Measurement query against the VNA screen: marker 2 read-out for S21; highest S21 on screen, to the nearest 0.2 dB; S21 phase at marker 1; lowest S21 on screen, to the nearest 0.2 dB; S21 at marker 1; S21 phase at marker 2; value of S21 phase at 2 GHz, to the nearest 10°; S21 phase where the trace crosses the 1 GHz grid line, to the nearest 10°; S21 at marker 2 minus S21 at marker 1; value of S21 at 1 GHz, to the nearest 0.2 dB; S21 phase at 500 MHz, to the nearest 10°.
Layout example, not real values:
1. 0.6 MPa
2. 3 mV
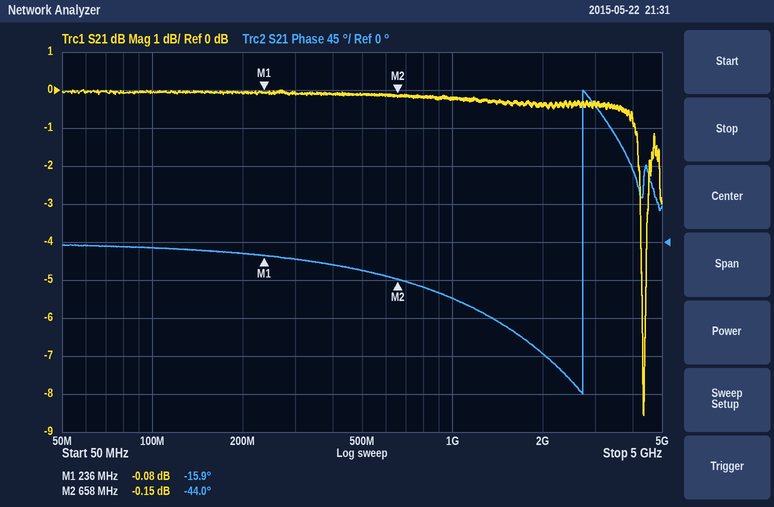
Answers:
1. -0.15 dB
2. 0.0 dB
3. -15.9°
4. -8.6 dB
5. -0.08 dB
6. -44.0°
7. -130°
8. -70°
9. -0.07 dB
10. -0.2 dB
11. -30°
